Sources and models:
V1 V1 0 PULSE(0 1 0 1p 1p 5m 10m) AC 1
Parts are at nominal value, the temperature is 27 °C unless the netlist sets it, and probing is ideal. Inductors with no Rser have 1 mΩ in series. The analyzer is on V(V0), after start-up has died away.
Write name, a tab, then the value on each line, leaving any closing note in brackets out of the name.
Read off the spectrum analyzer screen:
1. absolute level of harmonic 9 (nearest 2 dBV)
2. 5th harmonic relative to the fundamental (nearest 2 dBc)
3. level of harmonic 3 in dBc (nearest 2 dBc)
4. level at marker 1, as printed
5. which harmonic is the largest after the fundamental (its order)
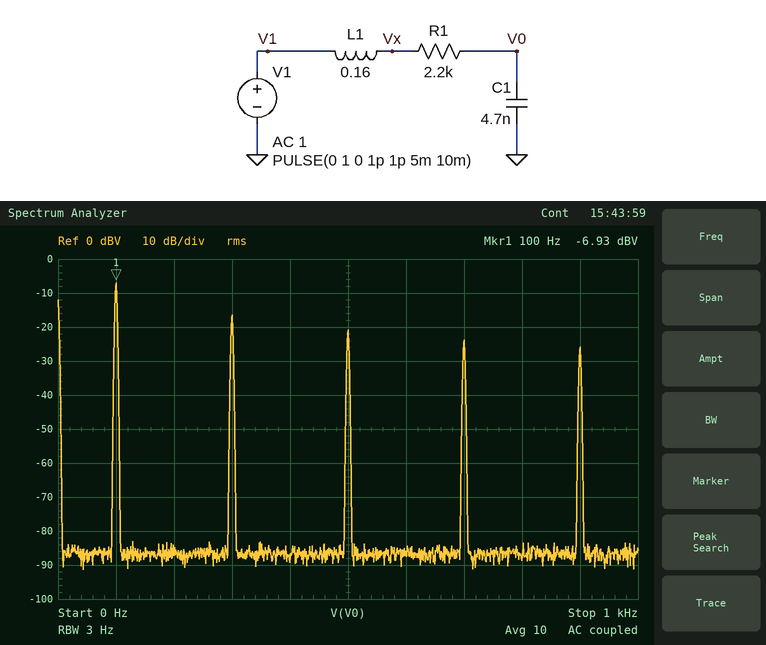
absolute level of harmonic 9	-26 dBV
5th harmonic relative to the fundamental	-14 dBc
level of harmonic 3 in dBc	-10 dBc
level at marker 1, as printed	-6.93 dBV
which harmonic is the largest after the fundamental	3
